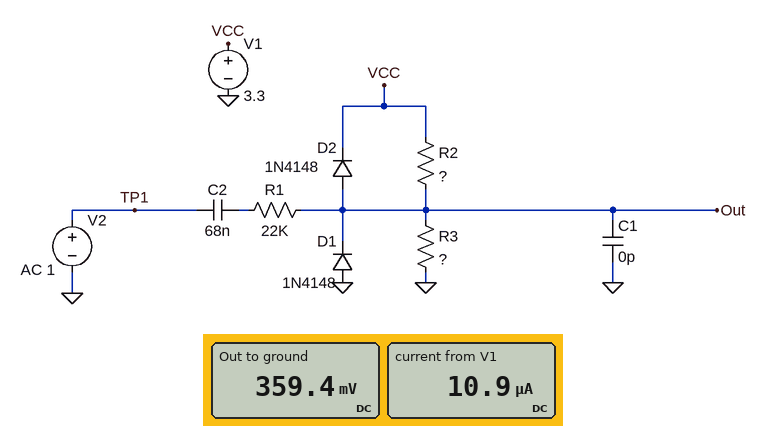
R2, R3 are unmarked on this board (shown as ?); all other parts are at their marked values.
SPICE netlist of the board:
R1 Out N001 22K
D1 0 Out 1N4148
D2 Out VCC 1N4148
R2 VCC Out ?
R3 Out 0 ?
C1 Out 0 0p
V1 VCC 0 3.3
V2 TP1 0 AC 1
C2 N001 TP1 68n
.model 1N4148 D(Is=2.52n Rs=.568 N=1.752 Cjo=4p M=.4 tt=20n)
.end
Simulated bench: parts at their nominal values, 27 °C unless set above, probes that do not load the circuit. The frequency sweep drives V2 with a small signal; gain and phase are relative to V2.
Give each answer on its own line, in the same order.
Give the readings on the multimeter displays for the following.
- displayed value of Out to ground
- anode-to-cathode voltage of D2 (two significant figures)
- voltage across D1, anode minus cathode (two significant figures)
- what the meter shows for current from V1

359.4 mV
-2.9 V
-360 mV
10.9 µA
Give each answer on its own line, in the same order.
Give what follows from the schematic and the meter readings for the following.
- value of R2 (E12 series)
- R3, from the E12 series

270 kΩ
33 kΩ
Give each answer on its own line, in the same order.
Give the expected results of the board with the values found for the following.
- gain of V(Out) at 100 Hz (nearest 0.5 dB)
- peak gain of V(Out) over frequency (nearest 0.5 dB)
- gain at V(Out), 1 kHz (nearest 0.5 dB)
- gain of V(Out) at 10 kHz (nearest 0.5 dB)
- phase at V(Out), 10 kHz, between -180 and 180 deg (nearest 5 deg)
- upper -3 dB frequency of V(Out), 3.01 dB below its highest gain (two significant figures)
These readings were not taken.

-5.5 dB
-5.0 dB
-5.0 dB
-5.0 dB
0 deg
2.2 MHz
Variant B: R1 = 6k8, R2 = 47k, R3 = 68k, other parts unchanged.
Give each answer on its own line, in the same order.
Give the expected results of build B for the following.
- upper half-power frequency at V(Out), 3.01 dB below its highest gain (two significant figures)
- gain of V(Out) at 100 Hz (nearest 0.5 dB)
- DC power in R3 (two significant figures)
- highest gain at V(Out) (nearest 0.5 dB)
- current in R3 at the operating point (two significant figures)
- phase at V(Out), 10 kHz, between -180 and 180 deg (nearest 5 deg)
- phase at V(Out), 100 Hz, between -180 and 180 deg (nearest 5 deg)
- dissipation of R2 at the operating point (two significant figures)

5.4 MHz
-3.5 dB
56 µW
-2.0 dB
29 µA
0 deg
35 deg
39 µW
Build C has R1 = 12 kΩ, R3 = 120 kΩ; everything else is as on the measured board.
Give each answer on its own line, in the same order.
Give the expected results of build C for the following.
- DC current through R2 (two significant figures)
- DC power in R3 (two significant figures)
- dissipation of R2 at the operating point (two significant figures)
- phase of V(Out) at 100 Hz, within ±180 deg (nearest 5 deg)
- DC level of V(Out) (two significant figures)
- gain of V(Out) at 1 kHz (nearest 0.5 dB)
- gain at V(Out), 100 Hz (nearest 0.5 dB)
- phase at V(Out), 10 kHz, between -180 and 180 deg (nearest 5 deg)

8.5 µA
8.6 µW
19 µW
15 deg
1.0 V
-1.0 dB
-1.5 dB
0 deg
